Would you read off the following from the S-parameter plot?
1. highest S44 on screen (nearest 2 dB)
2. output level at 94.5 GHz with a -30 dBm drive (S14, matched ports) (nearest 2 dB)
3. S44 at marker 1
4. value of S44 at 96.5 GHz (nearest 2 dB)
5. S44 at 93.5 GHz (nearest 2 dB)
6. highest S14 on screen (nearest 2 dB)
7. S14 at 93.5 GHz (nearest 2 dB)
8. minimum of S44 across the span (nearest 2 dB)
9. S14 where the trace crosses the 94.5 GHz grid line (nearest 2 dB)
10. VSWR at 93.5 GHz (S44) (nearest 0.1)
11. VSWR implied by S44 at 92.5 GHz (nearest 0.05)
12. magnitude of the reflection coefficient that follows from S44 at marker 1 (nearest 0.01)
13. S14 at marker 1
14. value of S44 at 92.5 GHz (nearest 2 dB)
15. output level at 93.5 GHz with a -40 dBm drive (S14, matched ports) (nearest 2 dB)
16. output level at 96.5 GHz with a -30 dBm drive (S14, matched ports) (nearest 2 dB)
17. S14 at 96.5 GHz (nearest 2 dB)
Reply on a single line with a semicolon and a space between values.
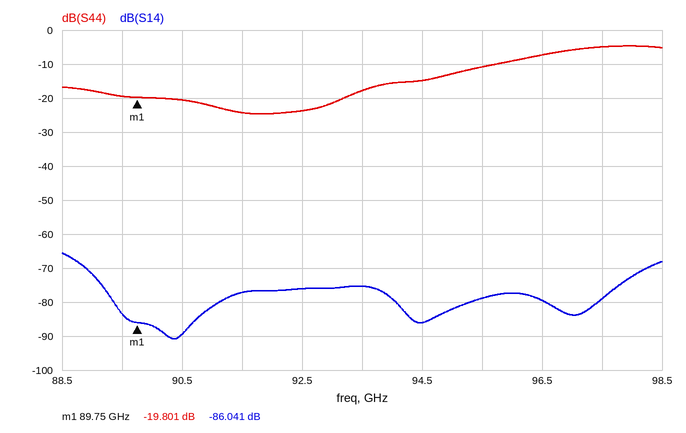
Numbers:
-4 dB; -116 dBm; -19.801 dB; -8 dB; -18 dB; -66 dB; -76 dB; -24 dB; -86 dB; 1.3; 1.15; 0.10; -86.041 dB; -24 dB; -116 dBm; -110 dBm; -80 dB
